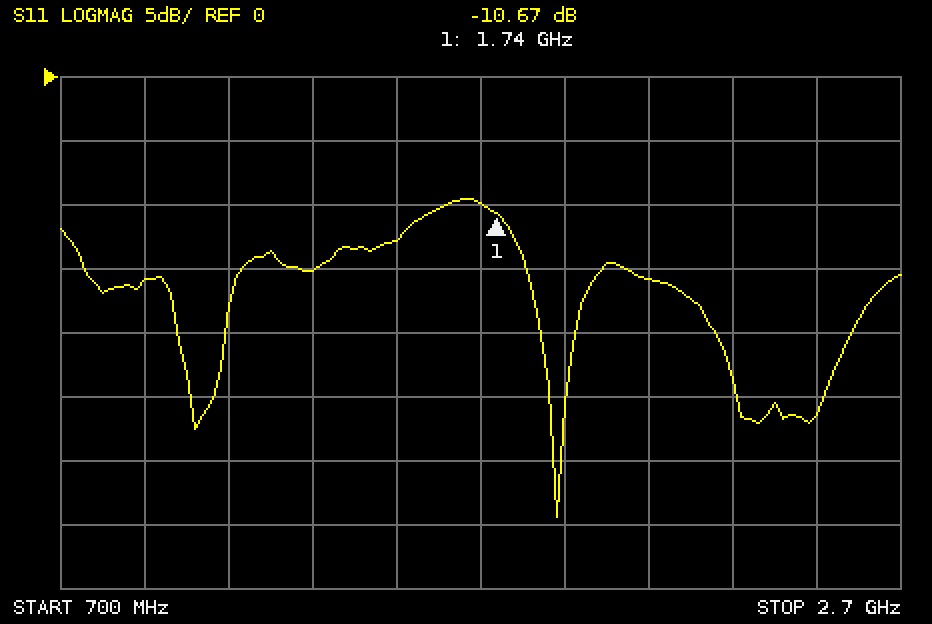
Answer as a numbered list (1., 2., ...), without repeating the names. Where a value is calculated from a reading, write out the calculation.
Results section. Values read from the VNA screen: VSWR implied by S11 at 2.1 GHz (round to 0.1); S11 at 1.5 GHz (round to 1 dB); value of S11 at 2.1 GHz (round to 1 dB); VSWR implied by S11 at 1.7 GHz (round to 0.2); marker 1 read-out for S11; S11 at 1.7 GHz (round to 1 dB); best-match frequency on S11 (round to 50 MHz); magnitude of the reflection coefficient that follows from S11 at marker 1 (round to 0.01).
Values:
1. |Γ| = 10^(-16/20) = 0.1585; VSWR = (1 + 0.1585)/(1 − 0.1585) ≈ 1.4
2. -13 dB
3. -16 dB
4. |Γ| = 10^(-10/20) = 0.3162; VSWR = (1 + 0.3162)/(1 − 0.3162) ≈ 1.92, so 2.0 to the nearest 0.2
5. -10.67 dB
6. -10 dB
7. 1.90 GHz
8. 10^(-10.67/20) ≈ 0.29
